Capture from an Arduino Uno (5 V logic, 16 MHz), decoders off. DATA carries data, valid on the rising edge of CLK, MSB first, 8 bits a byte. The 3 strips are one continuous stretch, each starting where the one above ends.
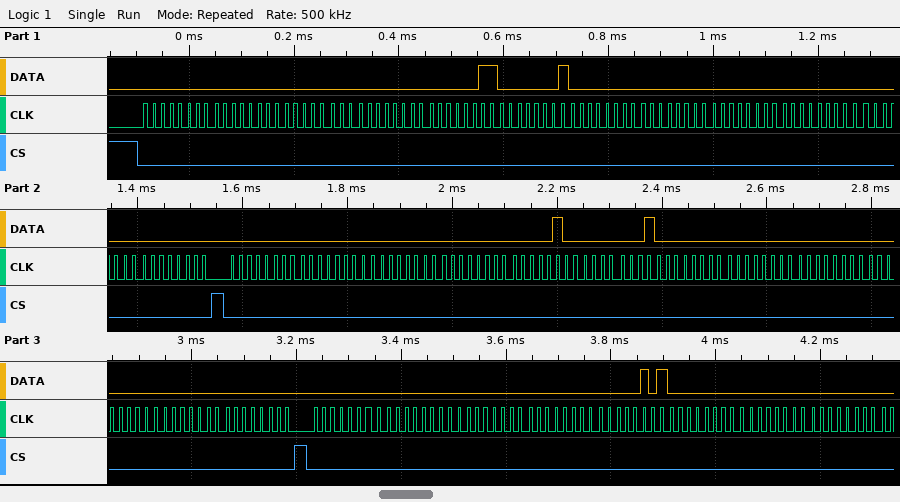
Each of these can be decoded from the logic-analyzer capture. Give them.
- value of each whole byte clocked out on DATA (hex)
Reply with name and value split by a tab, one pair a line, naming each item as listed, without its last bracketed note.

value of each whole byte clocked out on DATA	0x00 0x00 0x00 0x00 0x03 0x01 0x00 0x00 0x00 0x00 0x00 0x00 0x00 0x00 0x00 0x00 0x04 0x01 0x00 0x00 0x00 0x00 0x00 0x00 0x00 0x00 0x00 0x00 0x05 0x00 0x00 0x00
